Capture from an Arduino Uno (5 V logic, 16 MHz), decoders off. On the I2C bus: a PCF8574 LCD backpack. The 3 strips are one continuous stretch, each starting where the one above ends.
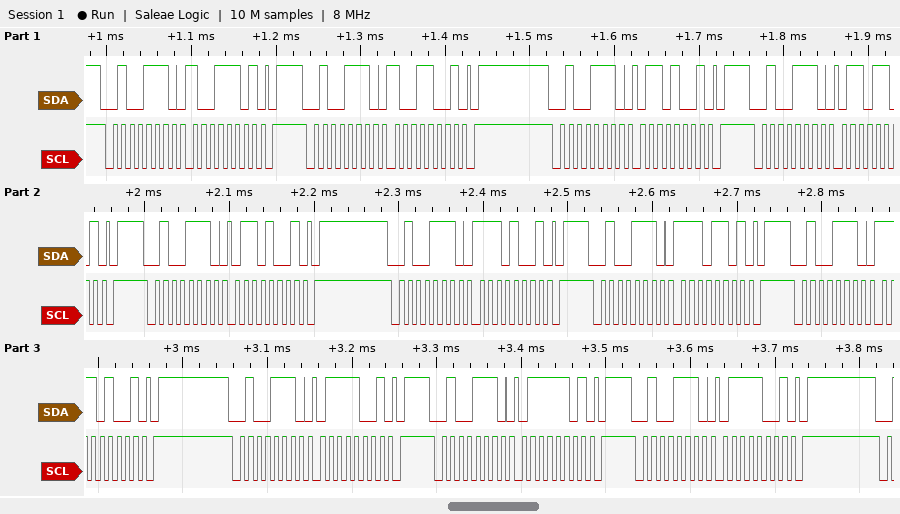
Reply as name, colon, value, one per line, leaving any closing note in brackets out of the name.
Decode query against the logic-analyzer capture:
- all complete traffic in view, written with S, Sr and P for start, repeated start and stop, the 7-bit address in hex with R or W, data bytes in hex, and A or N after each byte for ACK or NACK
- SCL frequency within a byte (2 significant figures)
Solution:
all complete traffic in view, written with S, Sr and P for start, repeated start and stop, the 7-bit address in hex with R or W, data bytes in hex, and A or N after each byte for ACK or NACK: S 27W A 9D A P S 27W A 99 A P S 27W A 69 A P S 27W A 6D A P S 27W A 69 A P S 27W A E9 A P S 27W A ED A P S 27W A E9 A P S 27W A 79 A P S 27W A 7D A P S 27W A 79 A P
SCL frequency within a byte: 100 kHz
